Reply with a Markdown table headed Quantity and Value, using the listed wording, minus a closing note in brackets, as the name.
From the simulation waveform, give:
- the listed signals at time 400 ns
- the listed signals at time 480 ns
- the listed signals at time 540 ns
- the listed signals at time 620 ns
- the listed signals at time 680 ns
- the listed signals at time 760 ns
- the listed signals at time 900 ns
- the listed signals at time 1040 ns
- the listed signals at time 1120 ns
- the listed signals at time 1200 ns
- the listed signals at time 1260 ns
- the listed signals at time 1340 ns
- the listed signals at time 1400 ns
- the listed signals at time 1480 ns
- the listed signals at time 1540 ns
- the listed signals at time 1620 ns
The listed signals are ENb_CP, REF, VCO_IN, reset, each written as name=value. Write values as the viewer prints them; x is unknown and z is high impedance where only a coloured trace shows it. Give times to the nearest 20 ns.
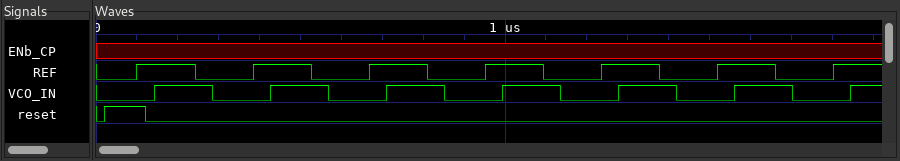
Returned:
| Quantity | Value |
|---|---|
| the listed signals at time 400 ns | ENb_CP=x, REF=1, VCO_IN=0, reset=0 |
| the listed signals at time 480 ns | ENb_CP=x, REF=1, VCO_IN=1, reset=0 |
| the listed signals at time 540 ns | ENb_CP=x, REF=0, VCO_IN=1, reset=0 |
| the listed signals at time 620 ns | ENb_CP=x, REF=0, VCO_IN=0, reset=0 |
| the listed signals at time 680 ns | ENb_CP=x, REF=1, VCO_IN=0, reset=0 |
| the listed signals at time 760 ns | ENb_CP=x, REF=1, VCO_IN=1, reset=0 |
| the listed signals at time 900 ns | ENb_CP=x, REF=0, VCO_IN=0, reset=0 |
| the listed signals at time 1040 ns | ENb_CP=x, REF=1, VCO_IN=1, reset=0 |
| the listed signals at time 1120 ns | ENb_CP=x, REF=0, VCO_IN=1, reset=0 |
| the listed signals at time 1200 ns | ENb_CP=x, REF=0, VCO_IN=0, reset=0 |
| the listed signals at time 1260 ns | ENb_CP=x, REF=1, VCO_IN=0, reset=0 |
| the listed signals at time 1340 ns | ENb_CP=x, REF=1, VCO_IN=1, reset=0 |
| the listed signals at time 1400 ns | ENb_CP=x, REF=0, VCO_IN=1, reset=0 |
| the listed signals at time 1480 ns | ENb_CP=x, REF=0, VCO_IN=0, reset=0 |
| the listed signals at time 1540 ns | ENb_CP=x, REF=1, VCO_IN=0, reset=0 |
| the listed signals at time 1620 ns | ENb_CP=x, REF=1, VCO_IN=1, reset=0 |
